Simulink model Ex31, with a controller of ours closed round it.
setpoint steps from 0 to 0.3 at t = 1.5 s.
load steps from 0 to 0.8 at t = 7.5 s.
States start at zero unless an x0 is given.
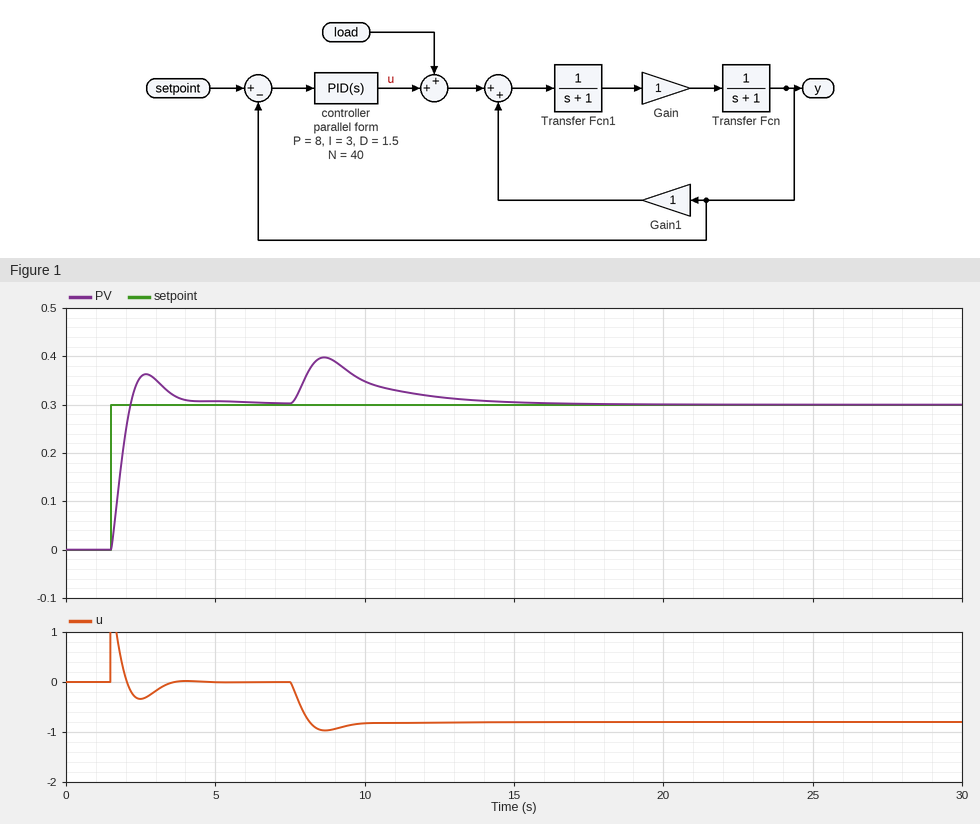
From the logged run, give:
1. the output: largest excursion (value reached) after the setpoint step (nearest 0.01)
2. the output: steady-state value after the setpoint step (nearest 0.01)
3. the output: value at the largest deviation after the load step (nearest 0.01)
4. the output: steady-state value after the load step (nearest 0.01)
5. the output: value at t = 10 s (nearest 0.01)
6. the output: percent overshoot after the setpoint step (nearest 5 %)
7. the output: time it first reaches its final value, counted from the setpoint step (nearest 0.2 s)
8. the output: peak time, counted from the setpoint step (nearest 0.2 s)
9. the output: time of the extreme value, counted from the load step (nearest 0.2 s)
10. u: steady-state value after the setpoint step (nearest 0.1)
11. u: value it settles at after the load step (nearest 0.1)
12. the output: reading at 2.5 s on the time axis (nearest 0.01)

0.36
0.30
0.40
0.30
0.35
20 %
0.6 s
1.2 s
1.2 s
0.0
-0.8
0.36
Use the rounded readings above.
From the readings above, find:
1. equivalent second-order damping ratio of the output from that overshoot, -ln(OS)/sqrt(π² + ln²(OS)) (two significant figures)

0.46
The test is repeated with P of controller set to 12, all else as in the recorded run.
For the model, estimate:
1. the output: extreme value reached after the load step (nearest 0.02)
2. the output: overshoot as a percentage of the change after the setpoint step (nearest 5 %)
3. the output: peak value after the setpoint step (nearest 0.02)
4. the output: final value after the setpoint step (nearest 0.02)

0.38
25 %
0.38
0.30
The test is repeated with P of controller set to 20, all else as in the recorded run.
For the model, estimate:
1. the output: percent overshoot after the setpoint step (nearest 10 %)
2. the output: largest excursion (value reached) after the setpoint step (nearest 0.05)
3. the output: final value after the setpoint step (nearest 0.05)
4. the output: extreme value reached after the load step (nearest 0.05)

30 %
0.40
0.30
0.35
